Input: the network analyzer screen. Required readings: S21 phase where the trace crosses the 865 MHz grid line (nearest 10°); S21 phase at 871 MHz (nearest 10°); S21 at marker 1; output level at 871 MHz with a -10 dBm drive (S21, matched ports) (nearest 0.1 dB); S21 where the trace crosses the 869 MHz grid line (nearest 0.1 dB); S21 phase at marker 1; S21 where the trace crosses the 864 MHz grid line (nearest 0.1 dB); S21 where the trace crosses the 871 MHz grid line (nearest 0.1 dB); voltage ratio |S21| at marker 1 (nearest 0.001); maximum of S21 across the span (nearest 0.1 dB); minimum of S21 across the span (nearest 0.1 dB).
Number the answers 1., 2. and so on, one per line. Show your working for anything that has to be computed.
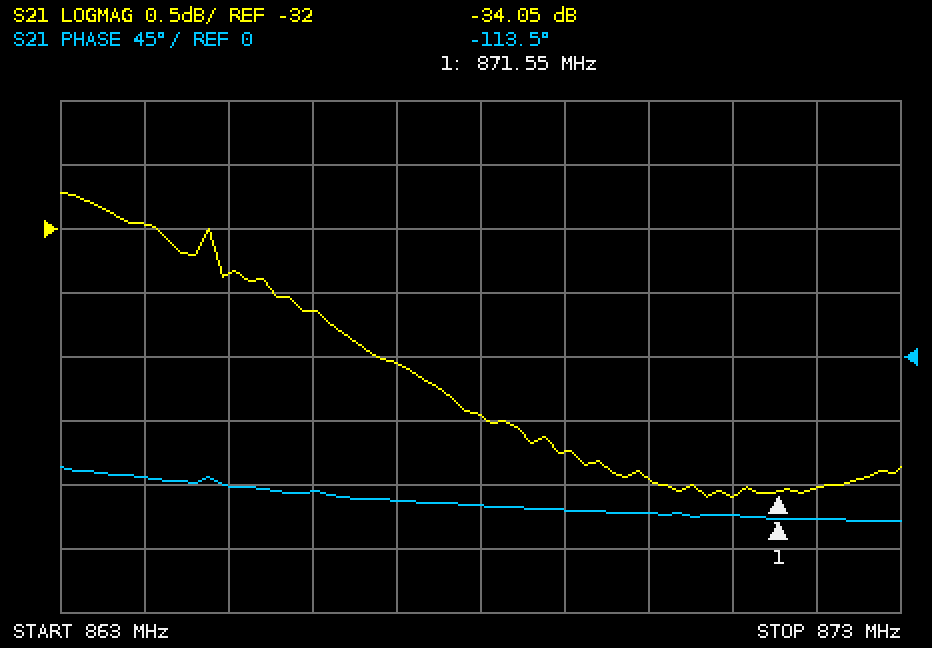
1. -90°
2. -110°
3. -34.05 dB
4. -10 dBm + (-34.1 dB) = -44.1 dBm
5. -33.7 dB
6. -113.5°
7. -32.0 dB
8. -34.1 dB
9. 10^(-34.05/20) ≈ 0.020
10. -31.7 dB
11. -34.1 dB
